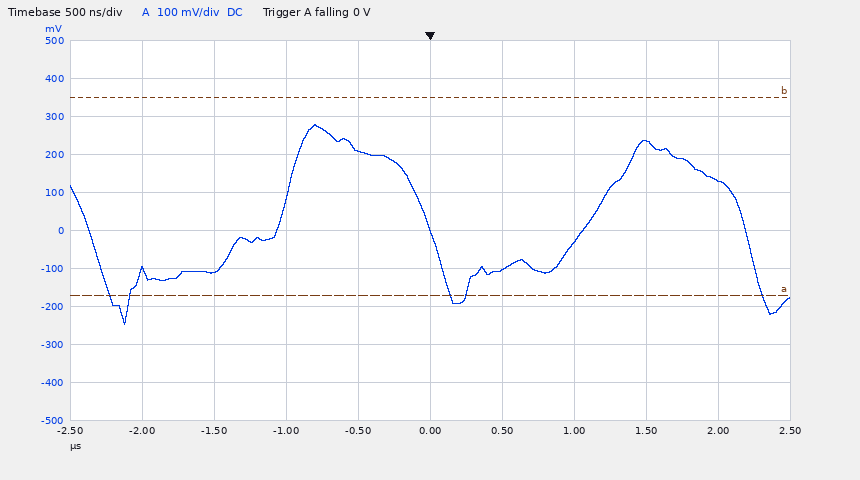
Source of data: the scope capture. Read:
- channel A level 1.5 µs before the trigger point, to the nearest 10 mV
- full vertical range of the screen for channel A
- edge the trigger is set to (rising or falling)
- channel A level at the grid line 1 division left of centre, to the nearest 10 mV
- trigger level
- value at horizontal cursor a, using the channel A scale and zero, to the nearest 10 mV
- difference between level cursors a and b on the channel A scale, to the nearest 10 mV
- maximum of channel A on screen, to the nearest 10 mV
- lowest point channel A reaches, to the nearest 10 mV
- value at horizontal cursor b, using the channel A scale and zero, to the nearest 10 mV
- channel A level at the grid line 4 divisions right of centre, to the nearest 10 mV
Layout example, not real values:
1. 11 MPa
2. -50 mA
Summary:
1. -110 mV
2. 1 V
3. falling
4. 210 mV
5. 0 V
6. -170 mV
7. 520 mV
8. 280 mV
9. -250 mV
10. 350 mV
11. 130 mV
